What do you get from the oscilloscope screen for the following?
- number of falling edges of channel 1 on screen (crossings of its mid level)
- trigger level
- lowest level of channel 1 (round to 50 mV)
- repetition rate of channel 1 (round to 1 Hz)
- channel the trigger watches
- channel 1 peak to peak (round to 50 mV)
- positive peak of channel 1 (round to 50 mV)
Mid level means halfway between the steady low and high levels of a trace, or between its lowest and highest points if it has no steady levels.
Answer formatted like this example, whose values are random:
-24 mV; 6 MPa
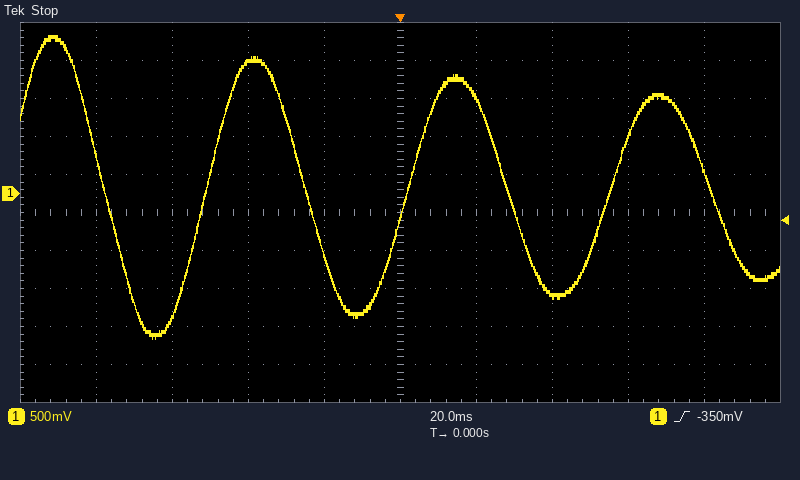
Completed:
4; -350 mV; -1.90 V; 19 Hz; channel 1; 4.00 V; 2.10 V
